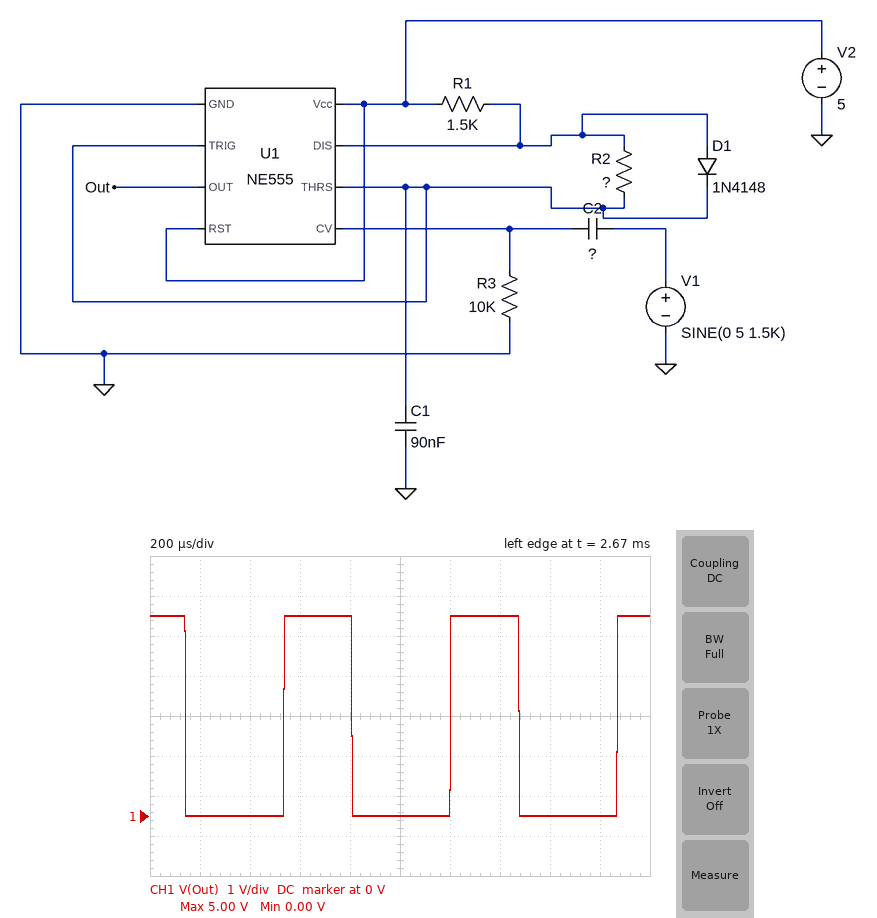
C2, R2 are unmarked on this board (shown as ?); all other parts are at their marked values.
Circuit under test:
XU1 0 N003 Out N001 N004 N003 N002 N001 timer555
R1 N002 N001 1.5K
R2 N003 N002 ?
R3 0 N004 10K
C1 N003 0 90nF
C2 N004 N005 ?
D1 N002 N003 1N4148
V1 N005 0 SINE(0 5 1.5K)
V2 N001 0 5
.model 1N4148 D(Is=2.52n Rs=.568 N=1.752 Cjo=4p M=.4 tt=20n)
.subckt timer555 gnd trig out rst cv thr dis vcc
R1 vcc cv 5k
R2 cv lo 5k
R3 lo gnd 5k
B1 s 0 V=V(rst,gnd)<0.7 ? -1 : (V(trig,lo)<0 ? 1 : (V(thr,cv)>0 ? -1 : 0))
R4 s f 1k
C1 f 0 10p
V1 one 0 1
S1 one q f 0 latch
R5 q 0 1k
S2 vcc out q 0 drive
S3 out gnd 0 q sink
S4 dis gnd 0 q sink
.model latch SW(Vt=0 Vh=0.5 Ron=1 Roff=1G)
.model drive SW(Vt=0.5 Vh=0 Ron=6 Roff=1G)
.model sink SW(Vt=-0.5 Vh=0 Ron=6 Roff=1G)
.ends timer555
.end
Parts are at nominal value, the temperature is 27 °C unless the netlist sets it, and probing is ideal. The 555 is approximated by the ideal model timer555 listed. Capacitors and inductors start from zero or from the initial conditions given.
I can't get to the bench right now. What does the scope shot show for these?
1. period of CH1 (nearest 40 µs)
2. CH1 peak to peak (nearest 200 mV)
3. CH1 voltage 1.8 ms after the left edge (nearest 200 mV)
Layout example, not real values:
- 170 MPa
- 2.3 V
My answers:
- 680 µs
- 5.0 V
- 0 V
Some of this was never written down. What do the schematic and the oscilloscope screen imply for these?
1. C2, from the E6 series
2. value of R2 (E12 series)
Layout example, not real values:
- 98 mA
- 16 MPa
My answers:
- 22 nF
- 3.3 kΩ
